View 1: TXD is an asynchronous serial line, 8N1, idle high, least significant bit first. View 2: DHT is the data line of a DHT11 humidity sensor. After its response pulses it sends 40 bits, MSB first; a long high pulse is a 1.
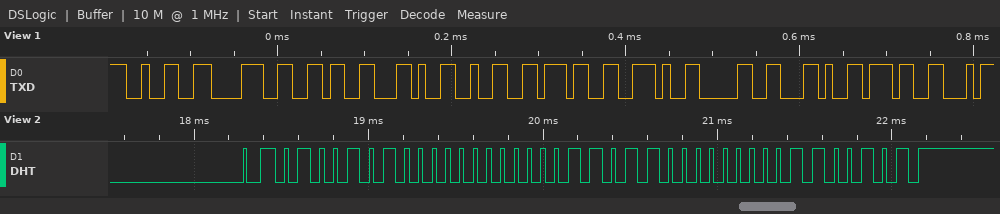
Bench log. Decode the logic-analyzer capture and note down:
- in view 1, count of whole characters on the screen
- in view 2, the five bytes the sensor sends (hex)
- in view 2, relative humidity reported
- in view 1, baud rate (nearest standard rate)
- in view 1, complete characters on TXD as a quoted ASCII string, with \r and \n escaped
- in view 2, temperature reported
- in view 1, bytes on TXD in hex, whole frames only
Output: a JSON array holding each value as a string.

["10", "4A 00 1B 00 65", "74 %", "115200 baud", "\"286,27.0,7\"", "27.0 °C", "32 38 36 2C 32 37 2E 30 2C 37"]
